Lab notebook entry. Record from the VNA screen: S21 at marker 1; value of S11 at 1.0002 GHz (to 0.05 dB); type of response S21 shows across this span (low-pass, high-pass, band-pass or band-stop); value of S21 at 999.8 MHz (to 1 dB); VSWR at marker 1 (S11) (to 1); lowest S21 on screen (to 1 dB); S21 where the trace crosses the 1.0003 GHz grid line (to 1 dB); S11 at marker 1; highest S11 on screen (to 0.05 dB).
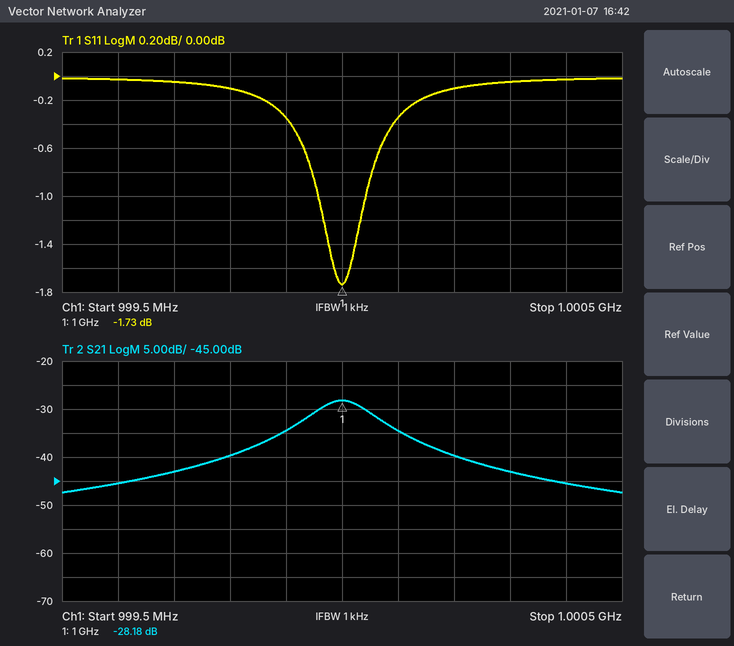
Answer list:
-28.18 dB
-0.10 dB
band-pass
-40 dB
10
-47 dB
-43 dB
-1.73 dB
0.00 dB
